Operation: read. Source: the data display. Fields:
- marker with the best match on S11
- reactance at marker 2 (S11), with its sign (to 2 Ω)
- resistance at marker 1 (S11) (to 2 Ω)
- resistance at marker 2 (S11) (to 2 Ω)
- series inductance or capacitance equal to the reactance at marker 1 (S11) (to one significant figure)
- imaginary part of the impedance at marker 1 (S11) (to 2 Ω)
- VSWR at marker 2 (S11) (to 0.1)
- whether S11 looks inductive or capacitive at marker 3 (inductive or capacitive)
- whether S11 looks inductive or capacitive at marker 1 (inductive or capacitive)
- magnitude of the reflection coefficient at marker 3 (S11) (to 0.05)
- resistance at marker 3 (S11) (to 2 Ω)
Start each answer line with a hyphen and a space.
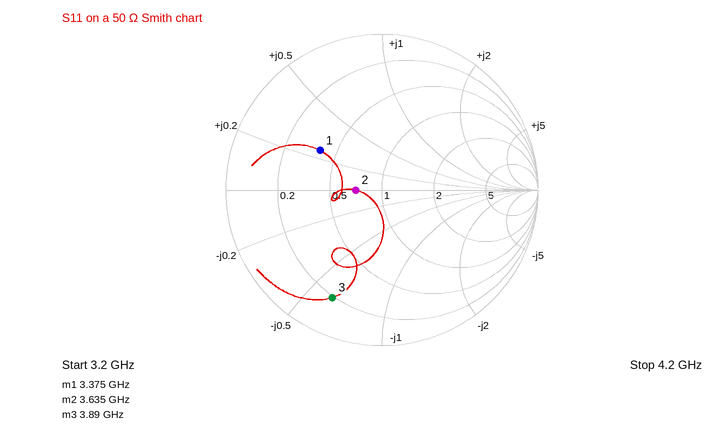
- marker 2
- 0 Ω
- 20 Ω
- 36 Ω
- 600 pH
- +12 Ω
- 1.4
- capacitive
- inductive
- 0.75
- 10 Ω
